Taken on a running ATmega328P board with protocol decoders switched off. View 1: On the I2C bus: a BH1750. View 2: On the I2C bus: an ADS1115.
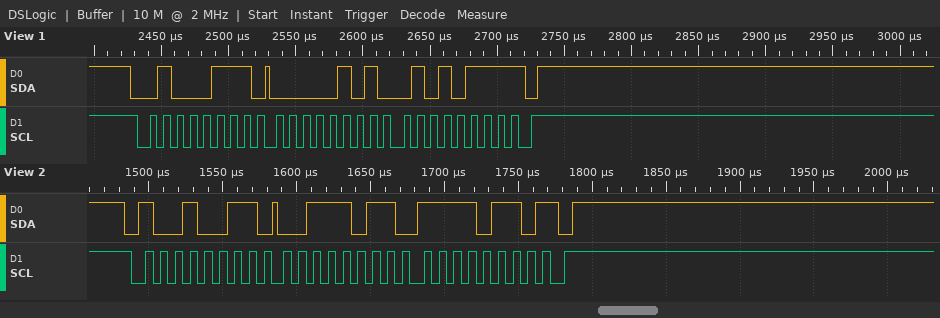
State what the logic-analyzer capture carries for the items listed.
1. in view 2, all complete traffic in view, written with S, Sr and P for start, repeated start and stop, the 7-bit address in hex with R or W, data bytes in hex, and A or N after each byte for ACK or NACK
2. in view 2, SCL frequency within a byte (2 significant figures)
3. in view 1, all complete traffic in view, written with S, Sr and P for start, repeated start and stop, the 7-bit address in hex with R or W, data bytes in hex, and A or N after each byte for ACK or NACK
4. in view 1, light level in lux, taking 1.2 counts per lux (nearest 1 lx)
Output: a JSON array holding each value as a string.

["S 49R A 3B A F6 N P", "100 kHz", "S 23R A 05 A 57 N P", "1139 lx"]
